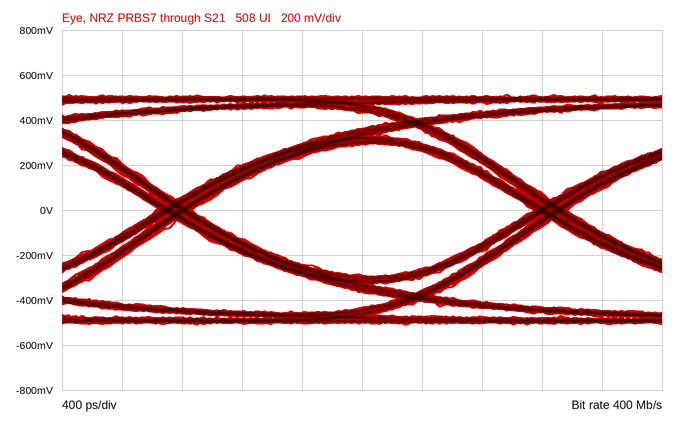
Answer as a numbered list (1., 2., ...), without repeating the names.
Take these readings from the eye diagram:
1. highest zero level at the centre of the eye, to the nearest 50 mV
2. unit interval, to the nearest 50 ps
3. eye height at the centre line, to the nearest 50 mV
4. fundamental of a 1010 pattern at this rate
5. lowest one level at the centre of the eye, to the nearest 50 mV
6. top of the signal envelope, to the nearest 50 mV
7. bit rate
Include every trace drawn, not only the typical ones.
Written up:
1. -300 mV
2. 2.50 ns
3. 600 mV
4. 200 MHz
5. 300 mV
6. 500 mV
7. 400 Mb/s
